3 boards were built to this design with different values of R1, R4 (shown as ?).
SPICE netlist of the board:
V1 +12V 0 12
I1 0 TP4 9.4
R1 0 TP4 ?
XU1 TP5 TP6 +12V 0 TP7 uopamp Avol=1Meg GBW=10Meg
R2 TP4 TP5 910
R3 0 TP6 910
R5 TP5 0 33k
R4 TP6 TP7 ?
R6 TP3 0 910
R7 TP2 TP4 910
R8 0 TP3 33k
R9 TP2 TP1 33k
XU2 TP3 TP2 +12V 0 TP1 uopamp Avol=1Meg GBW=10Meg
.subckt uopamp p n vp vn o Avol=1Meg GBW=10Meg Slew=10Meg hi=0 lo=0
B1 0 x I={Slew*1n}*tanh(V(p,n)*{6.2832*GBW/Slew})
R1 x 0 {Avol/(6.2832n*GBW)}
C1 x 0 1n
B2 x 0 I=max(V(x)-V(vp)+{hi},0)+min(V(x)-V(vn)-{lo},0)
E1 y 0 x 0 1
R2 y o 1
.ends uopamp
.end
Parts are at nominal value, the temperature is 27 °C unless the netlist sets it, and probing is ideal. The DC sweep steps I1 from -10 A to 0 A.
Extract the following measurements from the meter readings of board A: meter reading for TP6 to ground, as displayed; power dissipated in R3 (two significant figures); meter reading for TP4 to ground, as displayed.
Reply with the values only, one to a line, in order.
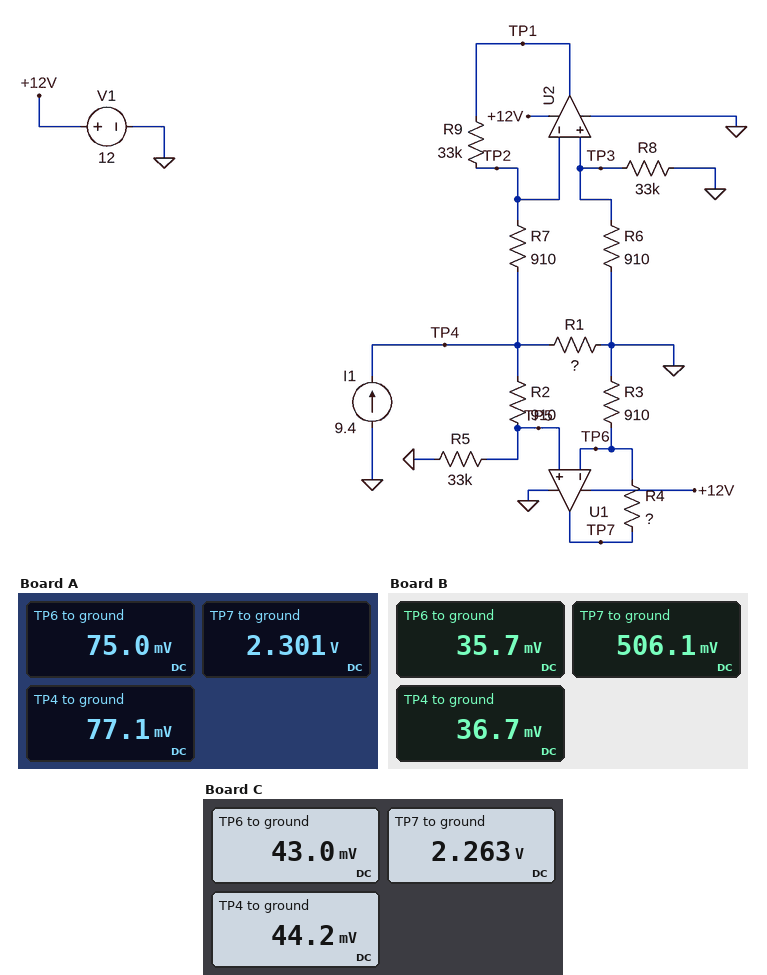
75.0 mV
6.2 µW
77.1 mV
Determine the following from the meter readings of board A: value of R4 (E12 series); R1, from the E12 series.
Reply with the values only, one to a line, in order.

27 kΩ
8.2 mΩ
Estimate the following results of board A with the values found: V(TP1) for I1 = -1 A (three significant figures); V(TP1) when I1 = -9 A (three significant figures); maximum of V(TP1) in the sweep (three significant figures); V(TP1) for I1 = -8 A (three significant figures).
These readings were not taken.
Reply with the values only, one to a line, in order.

297 mV
2.68 V
2.97 V
2.38 V
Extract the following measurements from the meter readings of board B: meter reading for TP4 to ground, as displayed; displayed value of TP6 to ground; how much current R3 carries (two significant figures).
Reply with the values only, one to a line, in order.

36.7 mV
35.7 mV
39 µA
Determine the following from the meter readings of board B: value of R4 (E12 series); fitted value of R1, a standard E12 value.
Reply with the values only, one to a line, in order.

12 kΩ
3.9 mΩ
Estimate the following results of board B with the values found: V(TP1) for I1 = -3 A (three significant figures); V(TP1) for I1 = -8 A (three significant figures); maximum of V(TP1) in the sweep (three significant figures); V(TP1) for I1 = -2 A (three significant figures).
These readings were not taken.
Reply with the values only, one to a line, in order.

424 mV
1.13 V
1.41 V
283 mV
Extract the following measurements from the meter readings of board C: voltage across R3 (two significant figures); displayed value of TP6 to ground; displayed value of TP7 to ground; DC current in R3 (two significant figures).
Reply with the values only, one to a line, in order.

43 mV
43.0 mV
2.263 V
47 µA
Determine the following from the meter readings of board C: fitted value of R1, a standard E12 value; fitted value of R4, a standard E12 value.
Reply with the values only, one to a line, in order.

4.7 mΩ
47 kΩ
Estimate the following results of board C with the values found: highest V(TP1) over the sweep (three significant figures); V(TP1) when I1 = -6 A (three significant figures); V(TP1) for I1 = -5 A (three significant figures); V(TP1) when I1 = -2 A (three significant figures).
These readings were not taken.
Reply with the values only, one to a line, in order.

1.70 V
1.02 V
852 mV
341 mV
